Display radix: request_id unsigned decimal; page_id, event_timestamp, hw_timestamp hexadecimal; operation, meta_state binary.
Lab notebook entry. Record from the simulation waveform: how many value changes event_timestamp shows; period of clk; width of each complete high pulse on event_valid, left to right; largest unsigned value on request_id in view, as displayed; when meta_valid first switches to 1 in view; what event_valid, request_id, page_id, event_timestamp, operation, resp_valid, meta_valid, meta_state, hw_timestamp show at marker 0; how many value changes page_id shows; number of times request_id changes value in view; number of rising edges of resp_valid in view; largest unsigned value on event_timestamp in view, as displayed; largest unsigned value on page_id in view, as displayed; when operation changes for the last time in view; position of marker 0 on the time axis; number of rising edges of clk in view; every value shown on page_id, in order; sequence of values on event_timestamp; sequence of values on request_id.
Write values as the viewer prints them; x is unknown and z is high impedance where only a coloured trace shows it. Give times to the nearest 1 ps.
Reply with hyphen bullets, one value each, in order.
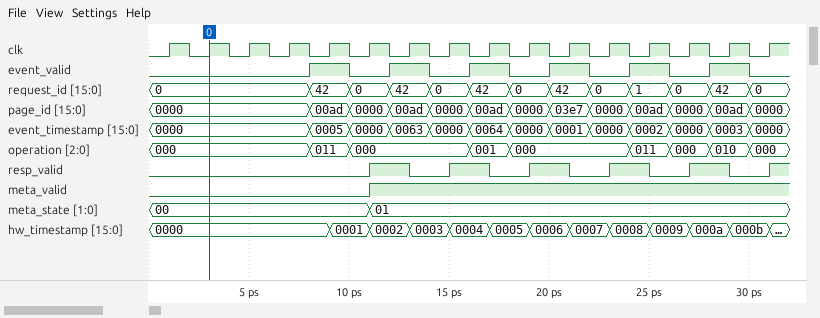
- 12
- 2 ps
- 2 ps, 2 ps, 2 ps, 2 ps, 2 ps, 2 ps
- 42
- 11 ps
- event_valid=0, request_id=0, page_id=0000, event_timestamp=0000, operation=000, resp_valid=0, meta_valid=0, meta_state=00, hw_timestamp=0000
- 12
- 12
- 6
- 0064
- 03e7
- 30 ps
- 3 ps
- 16
- 0000, 00ad, 0000, 00ad, 0000, 00ad, 0000, 03e7, 0000, 00ad, 0000, 00ad, 0000
- 0000, 0005, 0000, 0063, 0000, 0064, 0000, 0001, 0000, 0002, 0000, 0003, 0000
- 0, 42, 0, 42, 0, 42, 0, 42, 0, 1, 0, 42, 0
